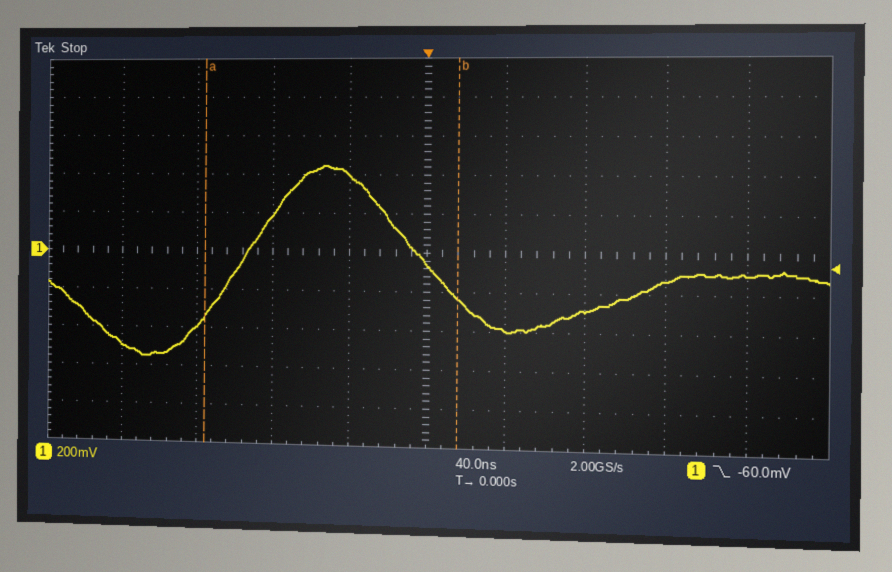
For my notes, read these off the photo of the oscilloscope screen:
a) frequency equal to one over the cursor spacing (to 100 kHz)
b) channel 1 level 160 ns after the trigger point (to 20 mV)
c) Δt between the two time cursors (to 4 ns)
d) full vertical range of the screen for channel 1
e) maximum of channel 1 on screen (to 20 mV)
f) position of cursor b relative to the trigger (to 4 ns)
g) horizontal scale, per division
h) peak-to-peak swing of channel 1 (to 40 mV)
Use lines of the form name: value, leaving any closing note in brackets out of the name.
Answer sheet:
frequency equal to one over the cursor spacing: 7.6 MHz
channel 1 level 160 ns after the trigger point: -100 mV
Δt between the two time cursors: 132 ns
full vertical range of the screen for channel 1: 2 V
maximum of channel 1 on screen: 440 mV
position of cursor b relative to the trigger: +16 ns
horizontal scale, per division: 40 ns
peak-to-peak swing of channel 1: 1.00 V
